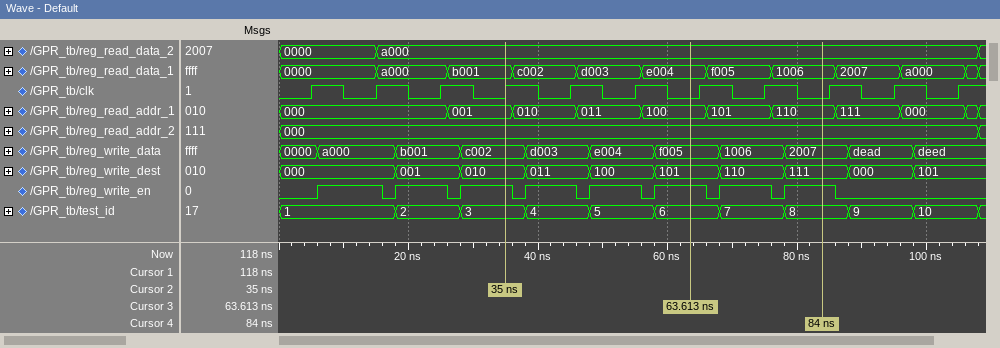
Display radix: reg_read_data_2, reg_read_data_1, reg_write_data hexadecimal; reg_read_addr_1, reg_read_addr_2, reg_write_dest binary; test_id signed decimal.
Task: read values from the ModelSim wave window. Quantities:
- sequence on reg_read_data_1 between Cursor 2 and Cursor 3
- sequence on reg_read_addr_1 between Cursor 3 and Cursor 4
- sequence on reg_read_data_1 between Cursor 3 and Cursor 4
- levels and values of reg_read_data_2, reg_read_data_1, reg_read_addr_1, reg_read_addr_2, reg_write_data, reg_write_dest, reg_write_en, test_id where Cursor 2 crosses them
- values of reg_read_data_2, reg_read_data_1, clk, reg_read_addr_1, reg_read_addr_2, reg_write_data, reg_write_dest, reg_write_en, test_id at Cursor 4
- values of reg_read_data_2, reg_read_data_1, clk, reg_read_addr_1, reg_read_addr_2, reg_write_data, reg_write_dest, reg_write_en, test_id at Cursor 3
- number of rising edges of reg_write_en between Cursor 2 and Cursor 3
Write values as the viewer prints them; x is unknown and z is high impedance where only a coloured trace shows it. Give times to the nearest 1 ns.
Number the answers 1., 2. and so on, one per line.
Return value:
1. b001, c002, d003, e004
2. 100, 101, 110
3. e004, f005, 1006
4. reg_read_data_2=a000, reg_read_data_1=b001, reg_read_addr_1=001, reg_read_addr_2=000, reg_write_data=c002, reg_write_dest=010, reg_write_en=1, test_id=3
5. reg_read_data_2=a000, reg_read_data_1=1006, clk=0, reg_read_addr_1=110, reg_read_addr_2=000, reg_write_data=2007, reg_write_dest=111, reg_write_en=1, test_id=8
6. reg_read_data_2=a000, reg_read_data_1=e004, clk=0, reg_read_addr_1=100, reg_read_addr_2=000, reg_write_data=f005, reg_write_dest=101, reg_write_en=1, test_id=6
7. 3
